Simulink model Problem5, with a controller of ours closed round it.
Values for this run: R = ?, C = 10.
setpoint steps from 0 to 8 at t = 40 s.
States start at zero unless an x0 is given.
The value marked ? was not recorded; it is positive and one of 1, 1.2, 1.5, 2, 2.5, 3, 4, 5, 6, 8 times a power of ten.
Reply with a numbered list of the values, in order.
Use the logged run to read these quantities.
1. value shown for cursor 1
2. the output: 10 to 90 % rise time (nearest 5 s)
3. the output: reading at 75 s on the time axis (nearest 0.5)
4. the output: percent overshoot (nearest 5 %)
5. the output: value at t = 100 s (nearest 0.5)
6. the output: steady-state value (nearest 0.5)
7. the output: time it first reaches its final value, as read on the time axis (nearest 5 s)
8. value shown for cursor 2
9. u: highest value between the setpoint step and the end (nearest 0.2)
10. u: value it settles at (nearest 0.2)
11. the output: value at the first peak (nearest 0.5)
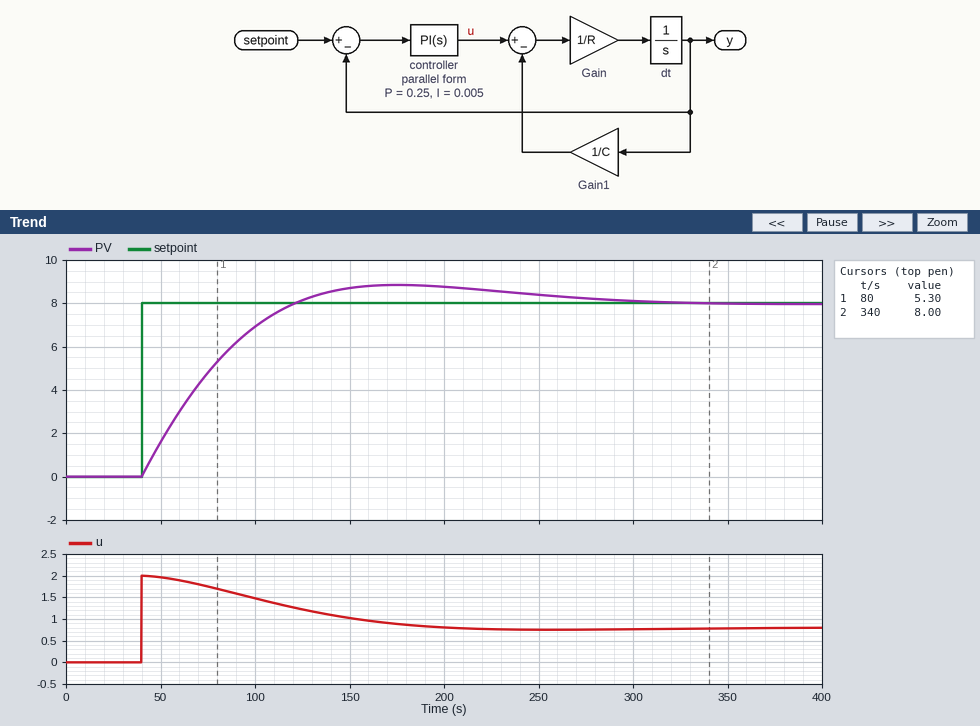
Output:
1. 5.30
2. 60 s
3. 5.0
4. 10 %
5. 7.0
6. 8.0
7. 120 s
8. 8.00
9. 2.0
10. 0.8
11. 9.0
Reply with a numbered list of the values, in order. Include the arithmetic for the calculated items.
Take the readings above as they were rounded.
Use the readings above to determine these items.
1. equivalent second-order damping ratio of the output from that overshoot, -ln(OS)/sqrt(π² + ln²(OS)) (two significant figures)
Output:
1. ln(0.1) = -2.303; 2.303 / sqrt(9.870 + 5.302) = 0.59
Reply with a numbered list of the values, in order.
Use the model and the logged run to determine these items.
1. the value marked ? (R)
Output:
1. 12
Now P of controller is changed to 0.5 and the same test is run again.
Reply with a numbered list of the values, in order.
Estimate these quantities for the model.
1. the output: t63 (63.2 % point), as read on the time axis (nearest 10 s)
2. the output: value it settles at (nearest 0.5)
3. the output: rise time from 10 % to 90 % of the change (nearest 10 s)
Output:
1. 60 s
2. 8.0
3. 50 s
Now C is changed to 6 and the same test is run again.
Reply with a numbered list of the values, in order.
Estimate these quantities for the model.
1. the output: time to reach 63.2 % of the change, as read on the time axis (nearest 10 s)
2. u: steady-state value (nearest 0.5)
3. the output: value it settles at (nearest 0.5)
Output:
1. 80 s
2. 1.5
3. 8.0
